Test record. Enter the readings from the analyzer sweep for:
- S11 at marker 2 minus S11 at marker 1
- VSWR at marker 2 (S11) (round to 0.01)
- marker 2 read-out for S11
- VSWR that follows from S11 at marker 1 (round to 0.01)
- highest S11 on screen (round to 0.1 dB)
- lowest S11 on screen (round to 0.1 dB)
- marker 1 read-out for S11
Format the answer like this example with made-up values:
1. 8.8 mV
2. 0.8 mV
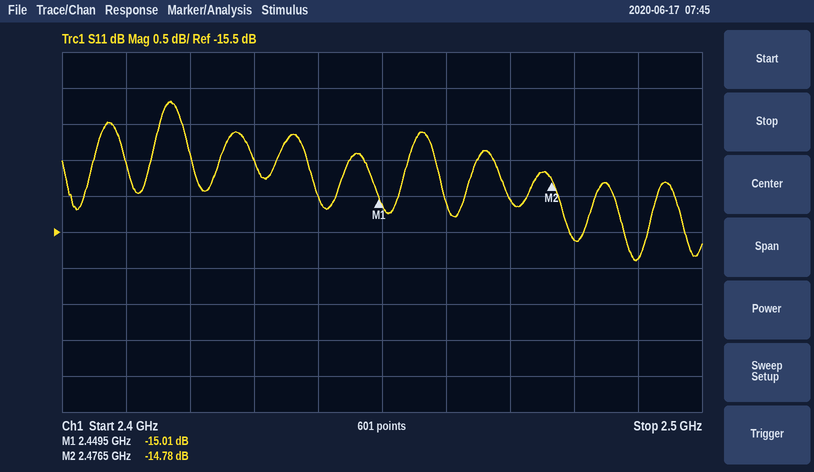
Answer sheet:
1. 0.23 dB
2. 1.45
3. -14.78 dB
4. 1.43
5. -13.7 dB
6. -15.9 dB
7. -15.01 dB
